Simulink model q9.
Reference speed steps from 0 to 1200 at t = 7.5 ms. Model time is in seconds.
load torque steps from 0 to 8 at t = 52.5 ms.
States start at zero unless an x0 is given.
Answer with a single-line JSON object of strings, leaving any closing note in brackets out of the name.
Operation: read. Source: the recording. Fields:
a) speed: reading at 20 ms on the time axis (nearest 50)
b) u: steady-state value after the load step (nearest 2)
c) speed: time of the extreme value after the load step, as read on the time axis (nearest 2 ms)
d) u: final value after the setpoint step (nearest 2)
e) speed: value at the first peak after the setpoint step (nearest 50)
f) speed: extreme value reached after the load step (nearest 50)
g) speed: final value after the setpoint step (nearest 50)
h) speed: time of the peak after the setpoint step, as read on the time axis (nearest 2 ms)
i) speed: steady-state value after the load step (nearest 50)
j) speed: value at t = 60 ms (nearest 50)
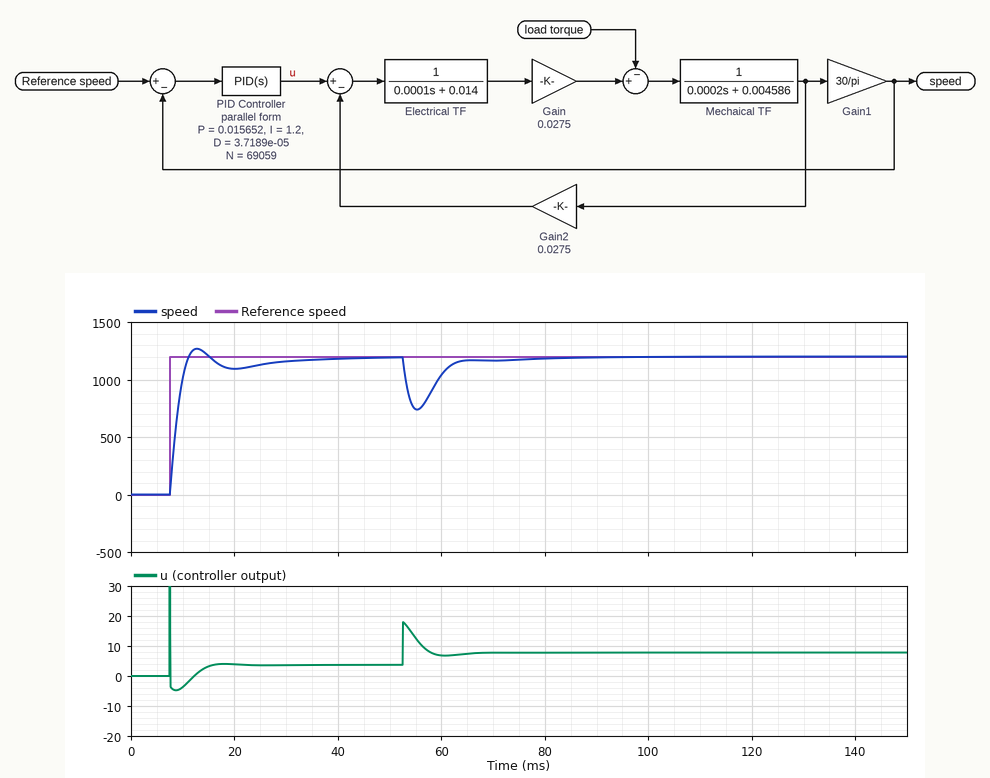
{"speed: reading at 20 ms on the time axis": "1100", "u: steady-state value after the load step": "8", "speed: time of the extreme value after the load step, as read on the time axis": "56 ms", "u: final value after the setpoint step": "4", "speed: value at the first peak after the setpoint step": "1250", "speed: extreme value reached after the load step": "750", "speed: final value after the setpoint step": "1200", "speed: time of the peak after the setpoint step, as read on the time axis": "12 ms", "speed: steady-state value after the load step": "1200", "speed: value at t = 60 ms": "1050"}
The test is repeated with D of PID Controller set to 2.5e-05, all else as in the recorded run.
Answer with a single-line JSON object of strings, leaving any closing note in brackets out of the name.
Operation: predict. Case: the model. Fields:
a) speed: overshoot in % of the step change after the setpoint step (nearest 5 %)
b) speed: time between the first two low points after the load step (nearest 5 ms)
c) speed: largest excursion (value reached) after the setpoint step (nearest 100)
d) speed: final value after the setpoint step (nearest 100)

{"speed: overshoot in % of the step change after the setpoint step": "15 %", "speed: time between the first two low points after the load step": "15 ms", "speed: largest excursion (value reached) after the setpoint step": "1400", "speed: final value after the setpoint step": "1200"}
